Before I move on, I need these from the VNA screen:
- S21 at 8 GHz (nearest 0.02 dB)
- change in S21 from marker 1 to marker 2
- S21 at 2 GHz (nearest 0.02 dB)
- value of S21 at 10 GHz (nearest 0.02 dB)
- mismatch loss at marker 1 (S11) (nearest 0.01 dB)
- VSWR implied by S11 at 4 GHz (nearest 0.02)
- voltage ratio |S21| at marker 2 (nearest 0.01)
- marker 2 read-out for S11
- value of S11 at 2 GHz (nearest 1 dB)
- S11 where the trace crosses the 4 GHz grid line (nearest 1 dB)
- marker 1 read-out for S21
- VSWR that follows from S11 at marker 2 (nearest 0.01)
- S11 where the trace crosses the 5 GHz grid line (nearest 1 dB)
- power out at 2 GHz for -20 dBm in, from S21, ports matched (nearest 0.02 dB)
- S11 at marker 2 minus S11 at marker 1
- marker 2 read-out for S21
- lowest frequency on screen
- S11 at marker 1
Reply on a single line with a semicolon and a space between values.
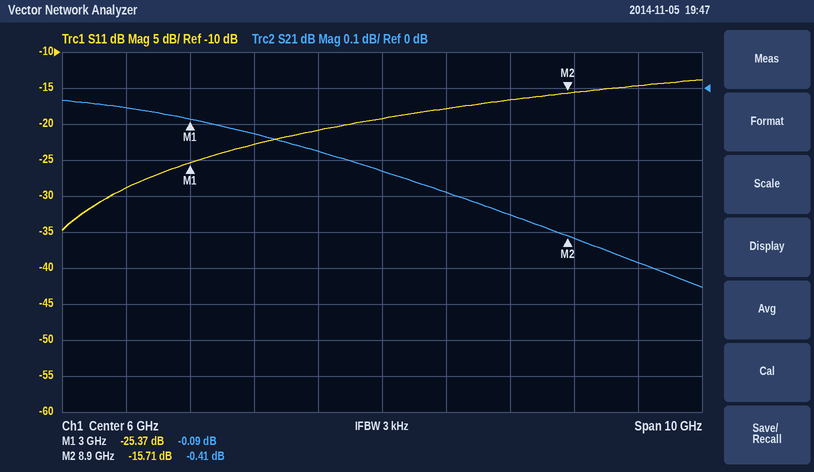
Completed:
-0.36 dB; -0.32 dB; -0.06 dB; -0.48 dB; 0.01 dB; 1.16; 0.95; -15.71 dB; -29 dB; -23 dB; -0.09 dB; 1.39; -21 dB; -20.06 dBm; 9.66 dB; -0.41 dB; 1 GHz; -25.37 dB
